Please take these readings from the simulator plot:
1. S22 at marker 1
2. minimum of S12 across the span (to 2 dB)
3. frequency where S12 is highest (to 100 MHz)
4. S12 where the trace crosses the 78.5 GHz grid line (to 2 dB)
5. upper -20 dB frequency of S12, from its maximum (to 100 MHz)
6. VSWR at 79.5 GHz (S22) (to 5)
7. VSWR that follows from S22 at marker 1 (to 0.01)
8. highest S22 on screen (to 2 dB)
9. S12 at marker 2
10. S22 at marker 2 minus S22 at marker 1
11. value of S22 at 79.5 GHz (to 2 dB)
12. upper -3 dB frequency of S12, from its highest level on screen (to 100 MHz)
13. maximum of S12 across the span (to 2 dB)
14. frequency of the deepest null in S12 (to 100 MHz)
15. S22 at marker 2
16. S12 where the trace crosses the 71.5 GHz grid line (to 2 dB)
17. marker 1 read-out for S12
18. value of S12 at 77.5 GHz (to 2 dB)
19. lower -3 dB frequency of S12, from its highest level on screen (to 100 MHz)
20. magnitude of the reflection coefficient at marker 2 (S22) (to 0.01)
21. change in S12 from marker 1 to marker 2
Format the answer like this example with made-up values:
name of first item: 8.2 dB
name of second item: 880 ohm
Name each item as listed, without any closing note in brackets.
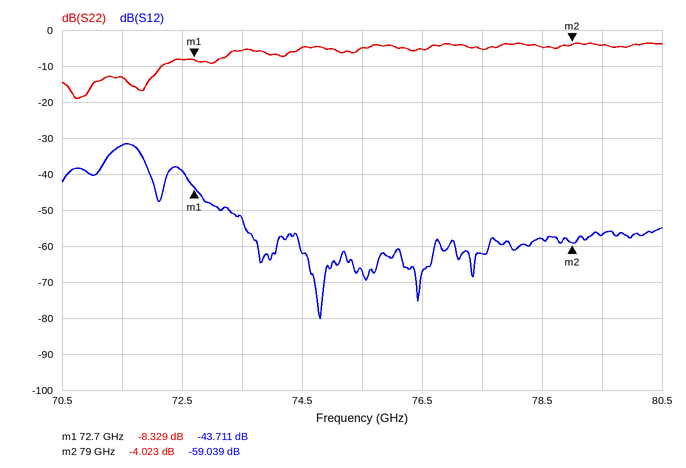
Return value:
S22 at marker 1: -8.329 dB
minimum of S12 across the span: -80 dB
frequency where S12 is highest: 71.6 GHz
S12 where the trace crosses the 78.5 GHz grid line: -58 dB
upper -20 dB frequency of S12, from its maximum: 73.4 GHz
VSWR at 79.5 GHz (S22): 5
VSWR that follows from S22 at marker 1: 2.24
highest S22 on screen: -4 dB
S12 at marker 2: -59.039 dB
S22 at marker 2 minus S22 at marker 1: 4.306 dB
value of S22 at 79.5 GHz: -4 dB
upper -3 dB frequency of S12, from its highest level on screen: 71.8 GHz
maximum of S12 across the span: -32 dB
frequency of the deepest null in S12: 74.8 GHz
S22 at marker 2: -4.023 dB
S12 where the trace crosses the 71.5 GHz grid line: -32 dB
marker 1 read-out for S12: -43.711 dB
value of S12 at 77.5 GHz: -62 dB
lower -3 dB frequency of S12, from its highest level on screen: 71.3 GHz
magnitude of the reflection coefficient at marker 2 (S22): 0.63
change in S12 from marker 1 to marker 2: -15.328 dB
